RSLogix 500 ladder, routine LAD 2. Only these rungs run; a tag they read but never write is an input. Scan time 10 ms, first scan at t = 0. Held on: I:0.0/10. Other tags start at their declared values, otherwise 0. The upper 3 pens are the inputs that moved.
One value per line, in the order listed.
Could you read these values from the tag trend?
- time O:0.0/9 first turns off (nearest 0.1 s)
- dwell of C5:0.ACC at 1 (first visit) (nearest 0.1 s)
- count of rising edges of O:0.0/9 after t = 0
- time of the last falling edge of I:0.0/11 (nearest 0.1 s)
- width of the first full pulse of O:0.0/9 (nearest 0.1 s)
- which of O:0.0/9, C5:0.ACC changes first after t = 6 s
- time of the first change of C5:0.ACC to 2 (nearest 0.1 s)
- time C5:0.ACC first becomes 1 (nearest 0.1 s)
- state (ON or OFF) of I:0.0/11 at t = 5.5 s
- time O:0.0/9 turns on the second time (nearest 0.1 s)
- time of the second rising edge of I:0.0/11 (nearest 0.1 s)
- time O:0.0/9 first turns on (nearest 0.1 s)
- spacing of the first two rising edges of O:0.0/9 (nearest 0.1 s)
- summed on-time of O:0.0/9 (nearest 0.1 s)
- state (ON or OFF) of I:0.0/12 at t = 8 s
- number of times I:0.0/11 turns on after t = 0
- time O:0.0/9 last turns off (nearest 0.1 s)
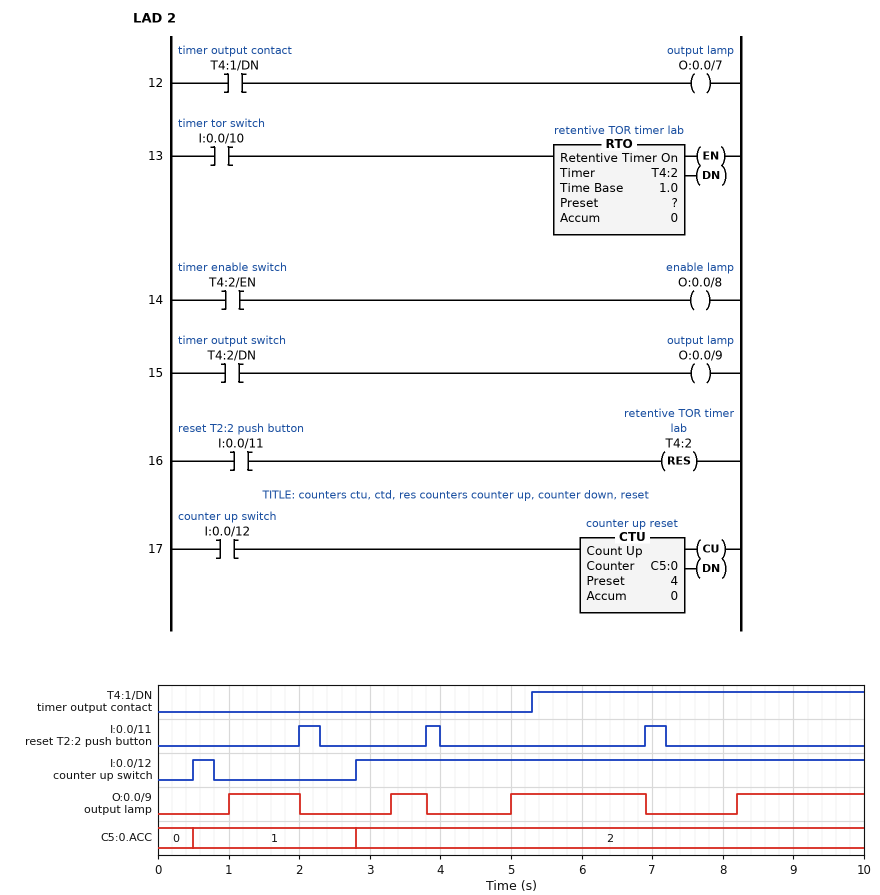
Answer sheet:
2.0 s
2.3 s
4
7.2 s
1.0 s
O:0.0/9
2.8 s
0.5 s
OFF
3.3 s
3.8 s
1.0 s
2.3 s
5.2 s
ON
3
6.9 s
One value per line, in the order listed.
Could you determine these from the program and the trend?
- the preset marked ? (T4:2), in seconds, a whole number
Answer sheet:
1 s
